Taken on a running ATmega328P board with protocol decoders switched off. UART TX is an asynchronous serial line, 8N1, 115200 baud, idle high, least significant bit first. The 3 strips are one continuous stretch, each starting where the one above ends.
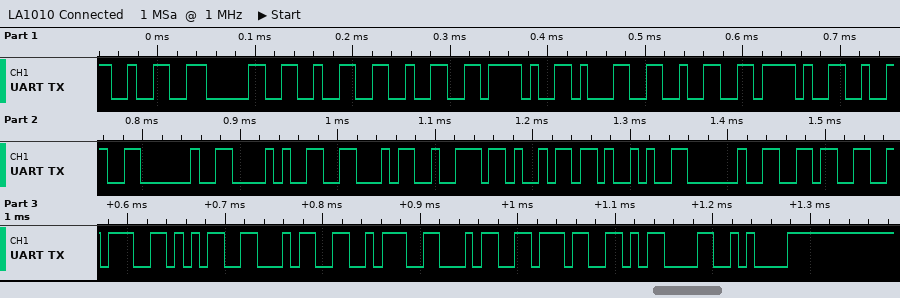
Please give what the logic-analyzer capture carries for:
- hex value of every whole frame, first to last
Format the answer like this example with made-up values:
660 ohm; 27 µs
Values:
32 30 32 32 2F 31 32 2F 32 20 28 46 72 69 29 20 36 3A 35 34 3A 34 37 0D 0A
